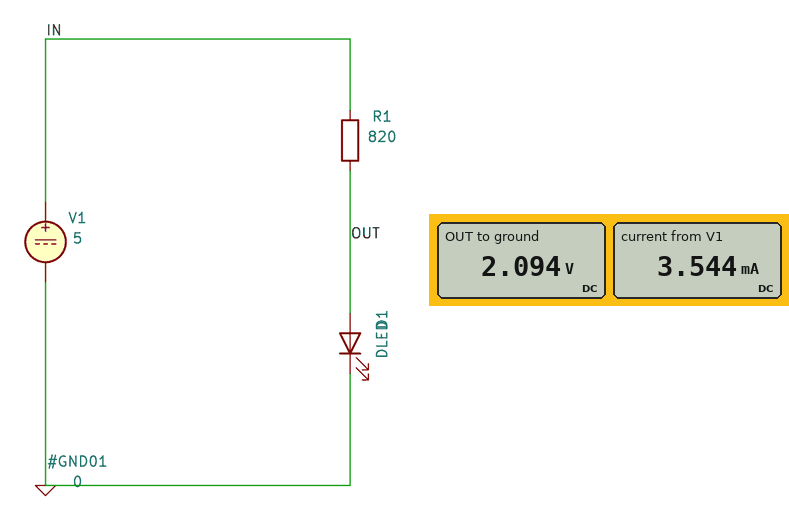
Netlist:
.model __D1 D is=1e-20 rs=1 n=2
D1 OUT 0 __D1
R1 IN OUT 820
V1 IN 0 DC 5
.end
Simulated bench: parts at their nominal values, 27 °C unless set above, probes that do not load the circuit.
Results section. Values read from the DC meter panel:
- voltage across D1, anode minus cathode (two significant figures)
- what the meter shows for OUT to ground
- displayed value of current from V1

2.1 V
2.094 V
3.544 mA
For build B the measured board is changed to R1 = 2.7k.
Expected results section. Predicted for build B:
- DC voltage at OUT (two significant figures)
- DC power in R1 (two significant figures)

2.0 V
3.3 mW
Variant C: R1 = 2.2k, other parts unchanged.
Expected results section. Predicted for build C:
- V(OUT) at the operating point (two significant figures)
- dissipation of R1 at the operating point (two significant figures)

2.0 V
4.0 mW
